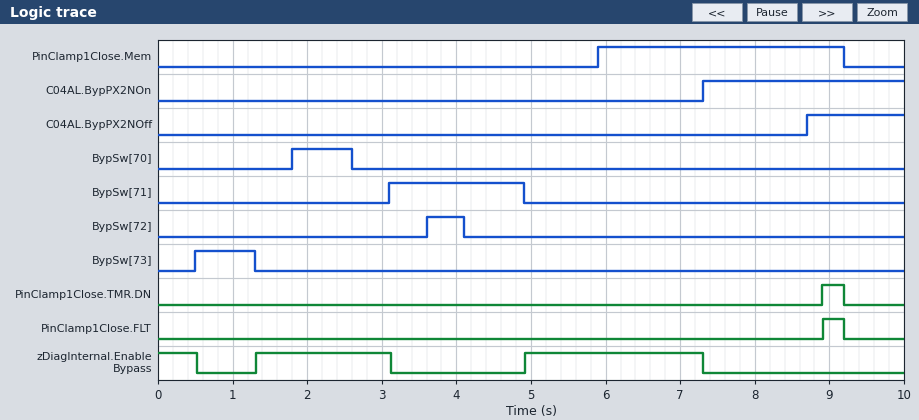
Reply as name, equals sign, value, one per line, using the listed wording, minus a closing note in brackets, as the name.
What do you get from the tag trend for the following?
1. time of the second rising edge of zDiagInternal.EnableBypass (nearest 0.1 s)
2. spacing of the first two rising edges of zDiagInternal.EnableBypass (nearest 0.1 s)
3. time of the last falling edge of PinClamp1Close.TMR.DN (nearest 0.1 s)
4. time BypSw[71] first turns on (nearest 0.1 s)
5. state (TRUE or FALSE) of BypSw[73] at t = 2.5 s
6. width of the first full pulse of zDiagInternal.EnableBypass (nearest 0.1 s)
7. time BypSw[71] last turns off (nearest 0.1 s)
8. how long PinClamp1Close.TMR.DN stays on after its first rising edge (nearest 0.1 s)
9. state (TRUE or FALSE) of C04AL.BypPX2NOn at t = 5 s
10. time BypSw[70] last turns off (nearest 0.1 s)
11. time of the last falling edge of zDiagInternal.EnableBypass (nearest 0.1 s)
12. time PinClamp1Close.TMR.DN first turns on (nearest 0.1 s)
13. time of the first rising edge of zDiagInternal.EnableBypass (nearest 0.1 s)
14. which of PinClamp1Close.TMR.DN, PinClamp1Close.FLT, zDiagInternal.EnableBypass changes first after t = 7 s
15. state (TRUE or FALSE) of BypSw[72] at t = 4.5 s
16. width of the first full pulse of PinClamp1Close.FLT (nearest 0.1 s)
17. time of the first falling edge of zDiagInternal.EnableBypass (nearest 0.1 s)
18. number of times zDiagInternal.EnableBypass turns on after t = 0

time of the second rising edge of zDiagInternal.EnableBypass = 4.9 s
spacing of the first two rising edges of zDiagInternal.EnableBypass = 3.6 s
time of the last falling edge of PinClamp1Close.TMR.DN = 9.2 s
time BypSw[71] first turns on = 3.1 s
state (TRUE or FALSE) of BypSw[73] at t = 2.5 s = FALSE
width of the first full pulse of zDiagInternal.EnableBypass = 1.8 s
time BypSw[71] last turns off = 4.9 s
how long PinClamp1Close.TMR.DN stays on after its first rising edge = 0.3 s
state (TRUE or FALSE) of C04AL.BypPX2NOn at t = 5 s = FALSE
time BypSw[70] last turns off = 2.6 s
time of the last falling edge of zDiagInternal.EnableBypass = 7.3 s
time PinClamp1Close.TMR.DN first turns on = 8.9 s
time of the first rising edge of zDiagInternal.EnableBypass = 1.3 s
which of PinClamp1Close.TMR.DN, PinClamp1Close.FLT, zDiagInternal.EnableBypass changes first after t = 7 s = zDiagInternal.EnableBypass
state (TRUE or FALSE) of BypSw[72] at t = 4.5 s = FALSE
width of the first full pulse of PinClamp1Close.FLT = 0.3 s
time of the first falling edge of zDiagInternal.EnableBypass = 0.5 s
number of times zDiagInternal.EnableBypass turns on after t = 0 = 2
